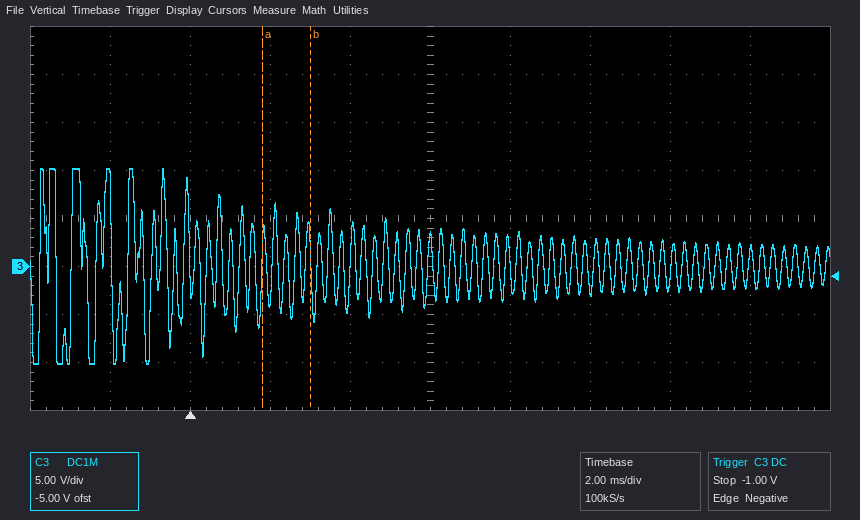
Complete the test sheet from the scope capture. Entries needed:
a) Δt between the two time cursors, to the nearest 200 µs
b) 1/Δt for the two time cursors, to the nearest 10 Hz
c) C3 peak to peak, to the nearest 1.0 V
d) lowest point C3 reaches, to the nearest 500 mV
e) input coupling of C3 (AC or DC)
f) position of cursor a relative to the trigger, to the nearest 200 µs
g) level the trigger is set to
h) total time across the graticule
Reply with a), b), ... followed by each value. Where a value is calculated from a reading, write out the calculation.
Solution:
a) 1.2 ms
b) 1 / 1.2 ms ≈ 830 Hz
c) 20.0 V
d) -10.0 V
e) DC
f) +1.8 ms
g) -1.00 V
h) 20 ms
